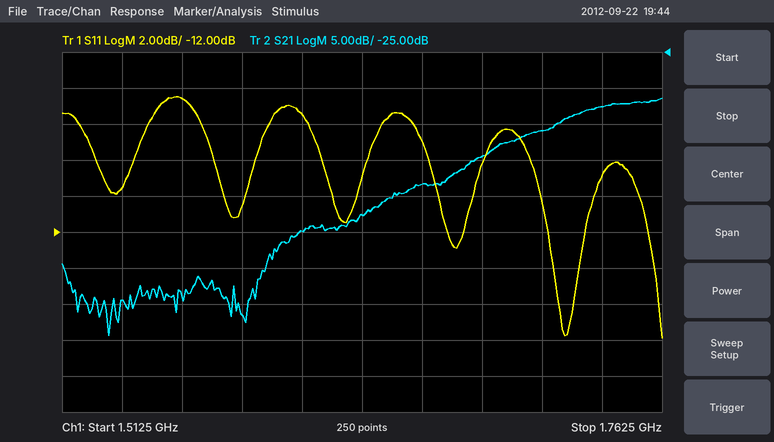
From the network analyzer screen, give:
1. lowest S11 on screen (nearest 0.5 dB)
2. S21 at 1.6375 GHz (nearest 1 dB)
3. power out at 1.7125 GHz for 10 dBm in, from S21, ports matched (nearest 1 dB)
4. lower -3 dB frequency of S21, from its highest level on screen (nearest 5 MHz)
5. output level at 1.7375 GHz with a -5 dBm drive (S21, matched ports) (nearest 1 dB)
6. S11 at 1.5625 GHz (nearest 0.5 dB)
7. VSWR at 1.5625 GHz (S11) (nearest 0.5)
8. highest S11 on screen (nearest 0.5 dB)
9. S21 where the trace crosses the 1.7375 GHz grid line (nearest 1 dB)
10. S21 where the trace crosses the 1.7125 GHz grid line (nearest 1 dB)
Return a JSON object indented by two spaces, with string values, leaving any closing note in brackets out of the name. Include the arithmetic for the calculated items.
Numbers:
{
  "lowest S11 on screen": "-18.0 dB",
  "S21 at 1.6375 GHz": "-48 dB",
  "power out at 1.7125 GHz for 10 dBm in, from S21, ports matched": "10 dBm + (-36 dB) = -26 dBm",
  "lower -3 dB frequency of S21, from its highest level on screen": "1.720 GHz",
  "output level at 1.7375 GHz with a -5 dBm drive (S21, matched ports)": "-5 dBm + (-33 dB) = -38 dBm",
  "S11 at 1.5625 GHz": "-4.5 dB",
  "VSWR at 1.5625 GHz (S11)": "|Γ| = 10^(-4.5/20) = 0.5957; VSWR = (1 + 0.5957)/(1 − 0.5957) ≈ 4.0",
  "highest S11 on screen": "-4.5 dB",
  "S21 where the trace crosses the 1.7375 GHz grid line": "-33 dB",
  "S21 where the trace crosses the 1.7125 GHz grid line": "-36 dB"
}
